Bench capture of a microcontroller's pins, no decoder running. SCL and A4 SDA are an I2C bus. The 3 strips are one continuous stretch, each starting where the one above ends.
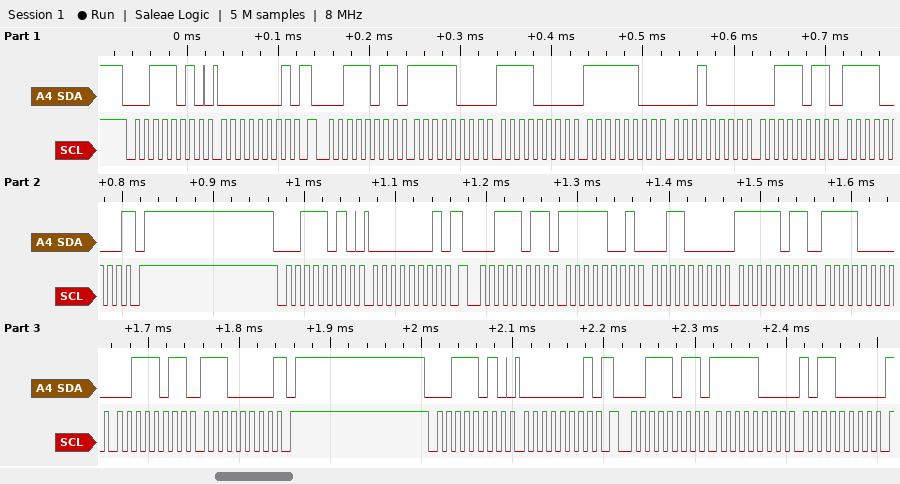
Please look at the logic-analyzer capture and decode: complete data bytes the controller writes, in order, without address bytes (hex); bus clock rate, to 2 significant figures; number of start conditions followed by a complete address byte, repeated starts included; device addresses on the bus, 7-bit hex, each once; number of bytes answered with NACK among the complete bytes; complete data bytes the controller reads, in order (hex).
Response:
01 01 01
100 kHz
6
0x1D
2
F8 F0 FC 10 3B F0 F9 30 FB F0 3B E0 F8 B0
